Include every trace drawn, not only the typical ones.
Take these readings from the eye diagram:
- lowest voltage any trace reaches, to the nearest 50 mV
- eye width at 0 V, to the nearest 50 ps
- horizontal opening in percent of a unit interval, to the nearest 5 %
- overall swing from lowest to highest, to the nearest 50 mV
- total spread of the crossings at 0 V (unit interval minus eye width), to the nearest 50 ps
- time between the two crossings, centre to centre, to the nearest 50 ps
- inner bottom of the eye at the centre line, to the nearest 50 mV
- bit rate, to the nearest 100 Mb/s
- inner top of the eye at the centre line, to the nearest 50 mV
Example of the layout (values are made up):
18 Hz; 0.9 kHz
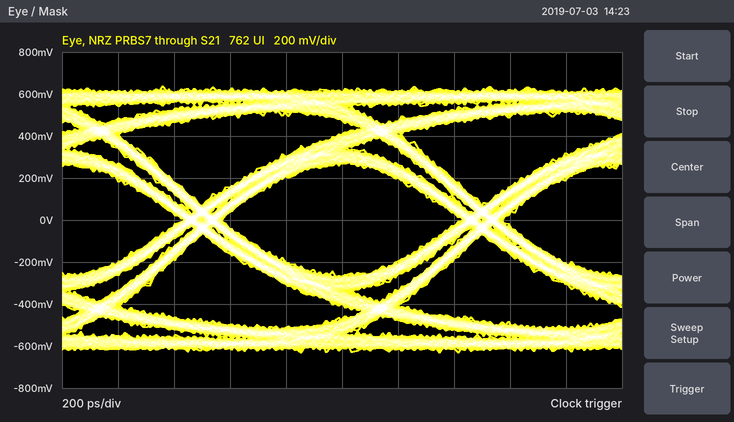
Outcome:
-650 mV; 850 ps; 85 %; 1.25 V; 150 ps; 1.00 ns; -250 mV; 1.0 Gb/s; 250 mV
